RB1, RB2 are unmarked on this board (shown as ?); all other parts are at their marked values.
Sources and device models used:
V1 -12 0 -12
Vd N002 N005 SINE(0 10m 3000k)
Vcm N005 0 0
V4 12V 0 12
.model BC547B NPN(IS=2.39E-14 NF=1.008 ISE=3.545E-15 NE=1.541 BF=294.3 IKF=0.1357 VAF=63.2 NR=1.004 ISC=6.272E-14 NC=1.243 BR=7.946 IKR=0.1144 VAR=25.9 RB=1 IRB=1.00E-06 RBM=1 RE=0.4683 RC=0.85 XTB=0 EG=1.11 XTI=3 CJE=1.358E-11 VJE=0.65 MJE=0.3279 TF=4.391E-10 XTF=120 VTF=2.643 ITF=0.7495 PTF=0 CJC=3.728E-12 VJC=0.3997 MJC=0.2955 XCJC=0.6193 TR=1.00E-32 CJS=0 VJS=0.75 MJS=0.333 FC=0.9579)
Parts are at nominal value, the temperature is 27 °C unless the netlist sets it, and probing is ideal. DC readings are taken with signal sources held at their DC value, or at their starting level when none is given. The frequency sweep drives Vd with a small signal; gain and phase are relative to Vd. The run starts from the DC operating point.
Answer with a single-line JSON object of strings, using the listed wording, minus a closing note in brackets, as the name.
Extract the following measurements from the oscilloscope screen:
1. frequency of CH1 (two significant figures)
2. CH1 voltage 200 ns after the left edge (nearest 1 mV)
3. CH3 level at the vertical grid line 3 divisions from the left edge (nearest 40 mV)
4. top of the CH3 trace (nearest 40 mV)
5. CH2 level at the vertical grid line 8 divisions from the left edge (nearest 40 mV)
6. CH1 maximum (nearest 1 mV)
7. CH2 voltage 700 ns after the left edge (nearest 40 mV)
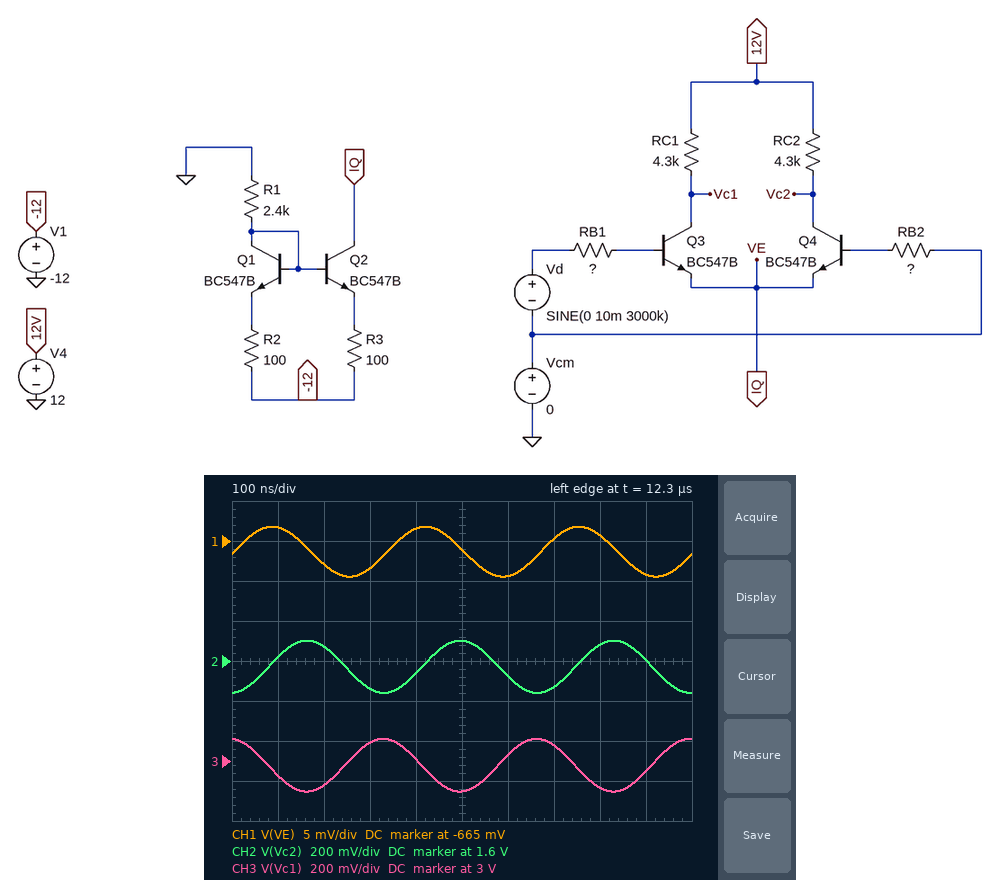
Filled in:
{"frequency of CH1": "3.0 MHz", "CH1 voltage 200 ns after the left edge": "-668 mV", "CH3 level at the vertical grid line 3 divisions from the left edge": "3.08 V", "top of the CH3 trace": "3.12 V", "CH2 level at the vertical grid line 8 divisions from the left edge": "1.68 V", "CH1 maximum": "-663 mV", "CH2 voltage 700 ns after the left edge": "1.48 V"}
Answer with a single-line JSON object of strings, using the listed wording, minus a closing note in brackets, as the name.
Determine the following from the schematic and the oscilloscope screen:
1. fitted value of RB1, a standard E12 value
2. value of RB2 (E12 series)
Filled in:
{"fitted value of RB1, a standard E12 value": "1.2 kΩ", "value of RB2": "470 Ω"}
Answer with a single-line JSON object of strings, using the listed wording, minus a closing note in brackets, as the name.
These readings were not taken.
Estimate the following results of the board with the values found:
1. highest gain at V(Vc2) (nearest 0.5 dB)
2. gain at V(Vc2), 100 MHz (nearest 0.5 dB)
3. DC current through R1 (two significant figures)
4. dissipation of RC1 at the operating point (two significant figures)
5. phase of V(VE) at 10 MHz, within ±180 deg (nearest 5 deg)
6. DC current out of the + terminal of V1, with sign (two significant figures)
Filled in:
{"highest gain at V(Vc2)": "42.0 dB", "gain at V(Vc2), 100 MHz": "-14.0 dB", "DC current through R1": "4.5 mA", "dissipation of RC1 at the operating point": "19 mW", "phase of V(VE) at 10 MHz, within ±180 deg": "-10 deg", "DC current out of the + terminal of V1, with sign": "-9.1 mA"}
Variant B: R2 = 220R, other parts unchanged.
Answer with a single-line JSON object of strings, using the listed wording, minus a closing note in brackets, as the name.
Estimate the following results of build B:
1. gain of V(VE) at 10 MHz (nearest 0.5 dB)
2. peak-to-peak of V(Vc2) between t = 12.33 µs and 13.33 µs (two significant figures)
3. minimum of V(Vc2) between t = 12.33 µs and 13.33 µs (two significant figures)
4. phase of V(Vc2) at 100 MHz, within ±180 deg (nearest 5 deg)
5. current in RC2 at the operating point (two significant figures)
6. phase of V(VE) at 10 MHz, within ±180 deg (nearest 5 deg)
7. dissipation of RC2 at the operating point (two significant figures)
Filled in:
{"gain of V(VE) at 10 MHz": "-12.5 dB", "peak-to-peak of V(Vc2) between t = 12.33 µs and 13.33 µs": "4.9 mV", "minimum of V(Vc2) between t = 12.33 µs and 13.33 µs": "-1.7 V", "phase of V(Vc2) at 100 MHz, within ±180 deg": "-20 deg", "current in RC2 at the operating point": "3.2 mA", "phase of V(VE) at 10 MHz, within ±180 deg": "-5 deg", "dissipation of RC2 at the operating point": "43 mW"}
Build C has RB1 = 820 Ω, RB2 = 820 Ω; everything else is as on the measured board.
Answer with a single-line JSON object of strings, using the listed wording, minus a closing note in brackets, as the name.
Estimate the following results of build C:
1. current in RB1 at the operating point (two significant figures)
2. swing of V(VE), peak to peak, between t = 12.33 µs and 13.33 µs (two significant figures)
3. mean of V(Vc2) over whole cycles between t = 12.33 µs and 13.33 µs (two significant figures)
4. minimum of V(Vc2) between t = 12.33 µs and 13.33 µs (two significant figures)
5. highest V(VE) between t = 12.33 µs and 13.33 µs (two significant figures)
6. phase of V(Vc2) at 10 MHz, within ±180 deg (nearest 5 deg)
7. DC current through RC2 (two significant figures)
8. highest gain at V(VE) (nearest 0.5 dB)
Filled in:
{"current in RB1 at the operating point": "7.8 µA", "swing of V(VE), peak to peak, between t = 12.33 µs and 13.33 µs": "10 mV", "mean of V(Vc2) over whole cycles between t = 12.33 µs and 13.33 µs": "2.3 V", "minimum of V(Vc2) between t = 12.33 µs and 13.33 µs": "2.1 V", "highest V(VE) between t = 12.33 µs and 13.33 µs": "-660 mV", "phase of V(Vc2) at 10 MHz, within ±180 deg": "-90 deg", "DC current through RC2": "2.3 mA", "highest gain at V(VE)": "-6.0 dB"}
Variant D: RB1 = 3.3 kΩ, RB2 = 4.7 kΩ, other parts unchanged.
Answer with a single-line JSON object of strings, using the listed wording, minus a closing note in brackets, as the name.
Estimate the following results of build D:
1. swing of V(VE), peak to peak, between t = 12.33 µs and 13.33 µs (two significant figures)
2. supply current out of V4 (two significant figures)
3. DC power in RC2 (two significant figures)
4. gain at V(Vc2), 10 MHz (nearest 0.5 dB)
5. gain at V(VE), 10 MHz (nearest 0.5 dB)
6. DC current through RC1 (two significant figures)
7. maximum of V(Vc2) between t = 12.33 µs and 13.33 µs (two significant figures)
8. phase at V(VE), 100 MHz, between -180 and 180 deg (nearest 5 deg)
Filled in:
{"swing of V(VE), peak to peak, between t = 12.33 µs and 13.33 µs": "11 mV", "supply current out of V4": "4.5 mA", "DC power in RC2": "19 mW", "gain at V(Vc2), 10 MHz": "-2.0 dB", "gain at V(VE), 10 MHz": "-6.5 dB", "DC current through RC1": "2.4 mA", "maximum of V(Vc2) between t = 12.33 µs and 13.33 µs": "3.1 V", "phase at V(VE), 100 MHz, between -180 and 180 deg": "-45 deg"}
